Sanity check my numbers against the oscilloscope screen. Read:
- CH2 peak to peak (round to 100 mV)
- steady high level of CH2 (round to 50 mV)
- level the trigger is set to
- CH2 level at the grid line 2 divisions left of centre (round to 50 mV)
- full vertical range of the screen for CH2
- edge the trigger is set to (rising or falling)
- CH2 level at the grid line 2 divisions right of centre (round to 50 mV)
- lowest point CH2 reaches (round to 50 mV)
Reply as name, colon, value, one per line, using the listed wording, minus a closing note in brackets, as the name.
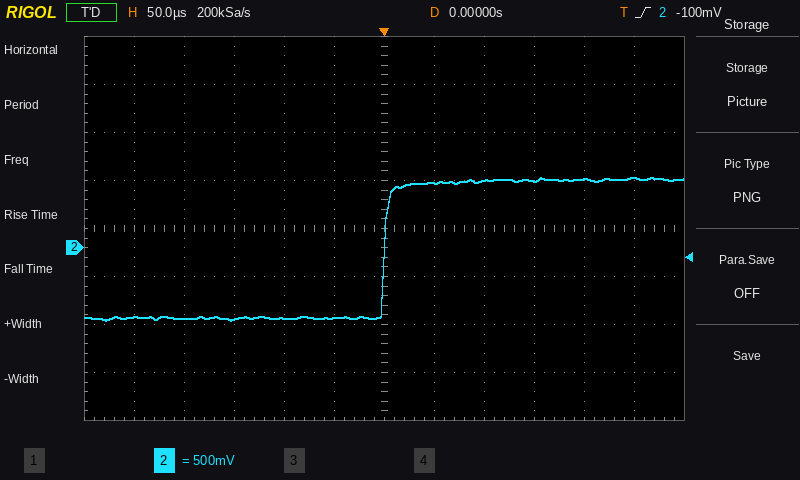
CH2 peak to peak: 1.50 V
steady high level of CH2: 700 mV
level the trigger is set to: -100 mV
CH2 level at the grid line 2 divisions left of centre: -750 mV
full vertical range of the screen for CH2: 4 V
edge the trigger is set to: rising
CH2 level at the grid line 2 divisions right of centre: 700 mV
lowest point CH2 reaches: -750 mV
